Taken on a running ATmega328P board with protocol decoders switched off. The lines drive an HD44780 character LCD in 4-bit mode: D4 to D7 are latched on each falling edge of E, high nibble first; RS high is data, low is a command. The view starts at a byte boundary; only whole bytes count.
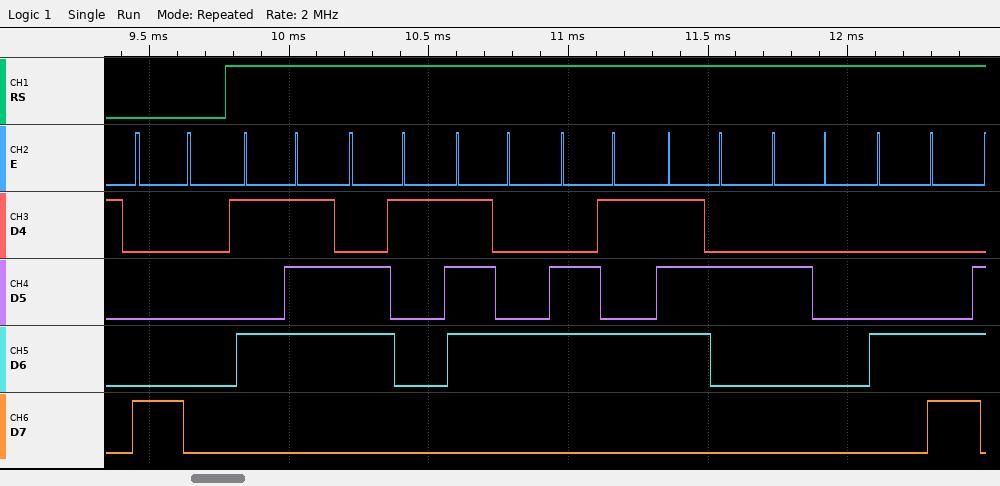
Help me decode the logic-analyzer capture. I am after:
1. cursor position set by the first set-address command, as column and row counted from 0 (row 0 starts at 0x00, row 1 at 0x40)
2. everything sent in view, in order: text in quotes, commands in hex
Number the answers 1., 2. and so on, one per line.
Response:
1. column 0, row 0
2. 0x80 "Water L"
